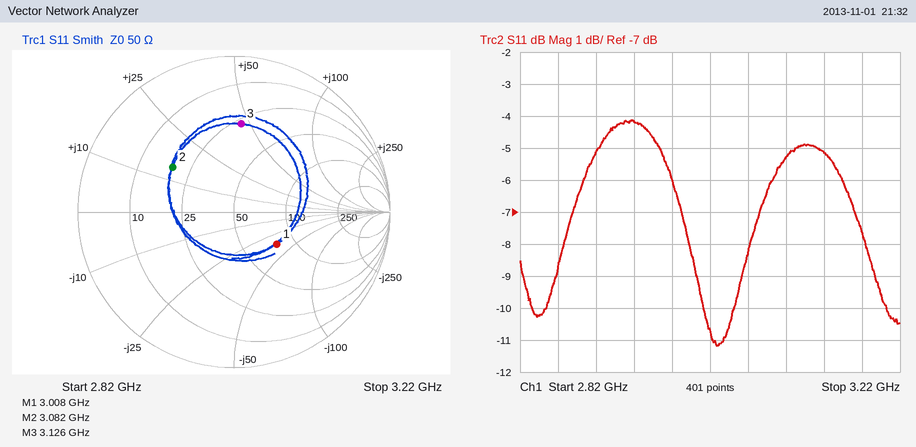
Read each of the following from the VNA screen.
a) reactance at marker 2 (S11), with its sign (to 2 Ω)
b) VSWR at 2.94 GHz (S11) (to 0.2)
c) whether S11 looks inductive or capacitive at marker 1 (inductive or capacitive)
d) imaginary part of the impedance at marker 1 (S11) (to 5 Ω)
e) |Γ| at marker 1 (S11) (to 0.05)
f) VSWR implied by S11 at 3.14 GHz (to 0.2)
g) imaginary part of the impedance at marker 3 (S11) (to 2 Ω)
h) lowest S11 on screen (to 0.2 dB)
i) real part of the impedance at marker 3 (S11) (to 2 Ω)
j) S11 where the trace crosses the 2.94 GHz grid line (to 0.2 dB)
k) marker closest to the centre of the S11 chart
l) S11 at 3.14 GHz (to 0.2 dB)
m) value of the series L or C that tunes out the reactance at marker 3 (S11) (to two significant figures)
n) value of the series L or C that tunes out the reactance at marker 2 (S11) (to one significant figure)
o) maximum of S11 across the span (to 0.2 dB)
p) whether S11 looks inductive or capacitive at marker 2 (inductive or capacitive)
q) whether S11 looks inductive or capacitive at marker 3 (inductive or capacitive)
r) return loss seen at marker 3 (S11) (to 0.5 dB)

+14 Ω
4.2
capacitive
-35 Ω
0.35
3.4
+46 Ω
-11.2 dB
28 Ω
-4.2 dB
marker 1
-5.2 dB
1.1 pF
4 pF
-4.2 dB
inductive
inductive
5.0 dB
